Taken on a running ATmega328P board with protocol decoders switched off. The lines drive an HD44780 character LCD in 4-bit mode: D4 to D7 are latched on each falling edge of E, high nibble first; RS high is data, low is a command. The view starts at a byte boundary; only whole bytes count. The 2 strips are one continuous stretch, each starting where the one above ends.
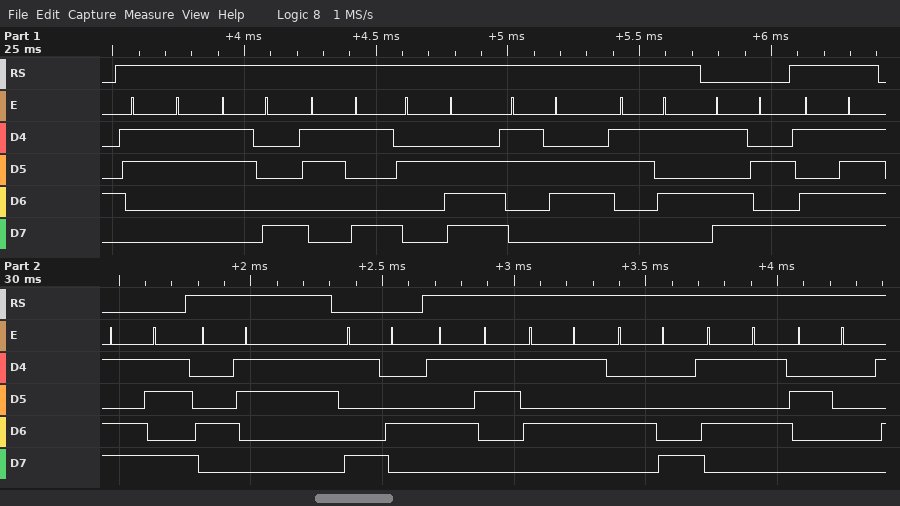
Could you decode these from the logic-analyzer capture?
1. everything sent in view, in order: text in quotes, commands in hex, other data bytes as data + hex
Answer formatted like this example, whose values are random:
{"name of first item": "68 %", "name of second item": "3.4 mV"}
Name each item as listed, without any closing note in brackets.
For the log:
{"everything sent in view, in order: text in quotes, commands in hex, other data bytes as data + hex": "\"389.65\" 0xDA data DF 0xDB \"C\" 0x94 \"SUHU \""}
